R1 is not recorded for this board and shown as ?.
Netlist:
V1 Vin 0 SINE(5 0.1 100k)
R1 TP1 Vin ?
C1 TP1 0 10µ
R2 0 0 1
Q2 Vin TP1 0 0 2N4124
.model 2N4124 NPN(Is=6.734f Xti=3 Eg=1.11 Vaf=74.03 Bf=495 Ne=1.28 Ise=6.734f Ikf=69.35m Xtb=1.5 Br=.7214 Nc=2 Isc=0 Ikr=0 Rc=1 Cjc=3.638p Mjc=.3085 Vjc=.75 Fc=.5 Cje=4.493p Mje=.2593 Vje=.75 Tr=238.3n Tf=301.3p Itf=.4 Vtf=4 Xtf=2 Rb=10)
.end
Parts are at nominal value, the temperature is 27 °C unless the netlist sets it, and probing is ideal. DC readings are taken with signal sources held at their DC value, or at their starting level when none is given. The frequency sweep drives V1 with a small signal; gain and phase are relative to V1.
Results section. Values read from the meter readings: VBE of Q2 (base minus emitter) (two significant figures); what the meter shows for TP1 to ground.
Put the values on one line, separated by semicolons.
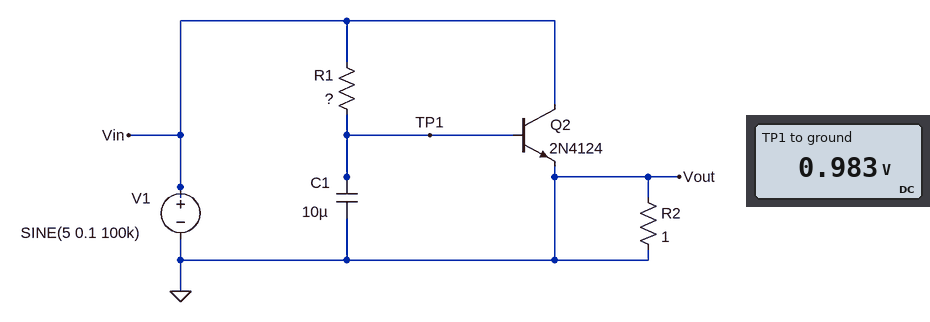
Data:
980 mV; 0.983 V
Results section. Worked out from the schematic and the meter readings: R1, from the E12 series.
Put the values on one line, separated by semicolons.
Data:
390 Ω
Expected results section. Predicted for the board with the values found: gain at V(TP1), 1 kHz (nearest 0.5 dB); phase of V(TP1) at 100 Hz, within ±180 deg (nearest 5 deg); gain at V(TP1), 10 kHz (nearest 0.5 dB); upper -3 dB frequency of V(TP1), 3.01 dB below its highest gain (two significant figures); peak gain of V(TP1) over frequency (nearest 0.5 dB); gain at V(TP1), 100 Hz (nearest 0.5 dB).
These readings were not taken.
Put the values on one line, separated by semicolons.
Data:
-32.0 dB; -5 deg; -48.0 dB; 1.3 kHz; -30.0 dB; -30.0 dB
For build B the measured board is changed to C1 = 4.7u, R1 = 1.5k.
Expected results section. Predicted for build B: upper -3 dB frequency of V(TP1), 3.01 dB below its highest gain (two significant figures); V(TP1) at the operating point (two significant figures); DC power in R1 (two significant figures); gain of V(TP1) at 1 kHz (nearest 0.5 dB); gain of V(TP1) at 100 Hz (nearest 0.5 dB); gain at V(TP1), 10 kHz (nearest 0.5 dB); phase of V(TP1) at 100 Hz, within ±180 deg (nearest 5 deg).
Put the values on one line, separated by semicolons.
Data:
1.7 kHz; 870 mV; 11 mW; -39.0 dB; -37.5 dB; -53.0 dB; -5 deg
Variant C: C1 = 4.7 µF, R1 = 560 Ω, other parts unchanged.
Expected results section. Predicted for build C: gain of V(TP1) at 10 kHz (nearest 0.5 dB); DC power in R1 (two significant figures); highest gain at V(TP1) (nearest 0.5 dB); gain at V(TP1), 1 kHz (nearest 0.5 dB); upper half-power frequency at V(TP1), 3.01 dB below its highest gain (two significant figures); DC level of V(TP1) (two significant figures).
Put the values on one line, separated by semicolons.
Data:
-44.5 dB; 29 mW; -32.5 dB; -33.0 dB; 2.5 kHz; 940 mV
